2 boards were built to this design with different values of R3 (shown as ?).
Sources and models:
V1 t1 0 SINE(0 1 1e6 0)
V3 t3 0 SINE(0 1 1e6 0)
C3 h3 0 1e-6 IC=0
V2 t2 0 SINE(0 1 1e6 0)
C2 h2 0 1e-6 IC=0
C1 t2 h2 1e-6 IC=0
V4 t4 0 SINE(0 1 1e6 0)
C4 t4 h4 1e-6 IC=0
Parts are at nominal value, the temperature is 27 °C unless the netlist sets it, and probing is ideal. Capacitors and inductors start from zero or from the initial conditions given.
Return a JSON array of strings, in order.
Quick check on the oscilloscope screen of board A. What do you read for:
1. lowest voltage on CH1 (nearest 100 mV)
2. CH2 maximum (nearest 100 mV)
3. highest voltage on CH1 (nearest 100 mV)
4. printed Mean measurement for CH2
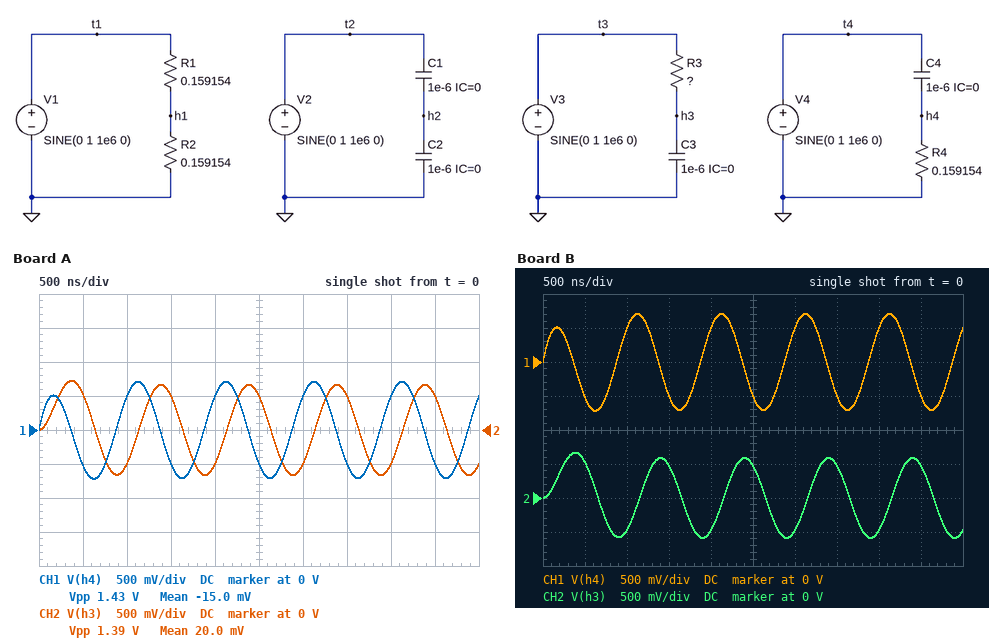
["-700 mV", "700 mV", "700 mV", "20.0 mV"]
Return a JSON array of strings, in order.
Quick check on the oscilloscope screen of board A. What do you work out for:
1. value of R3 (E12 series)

["0.18 Ω"]
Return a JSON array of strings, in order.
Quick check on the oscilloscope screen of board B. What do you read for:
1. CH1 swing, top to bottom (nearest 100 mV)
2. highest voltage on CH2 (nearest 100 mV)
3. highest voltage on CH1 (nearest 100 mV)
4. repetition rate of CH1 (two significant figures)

["1.4 V", "700 mV", "700 mV", "1.0 MHz"]
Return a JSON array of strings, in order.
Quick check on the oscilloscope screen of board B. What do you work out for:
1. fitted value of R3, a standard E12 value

["0.22 Ω"]
